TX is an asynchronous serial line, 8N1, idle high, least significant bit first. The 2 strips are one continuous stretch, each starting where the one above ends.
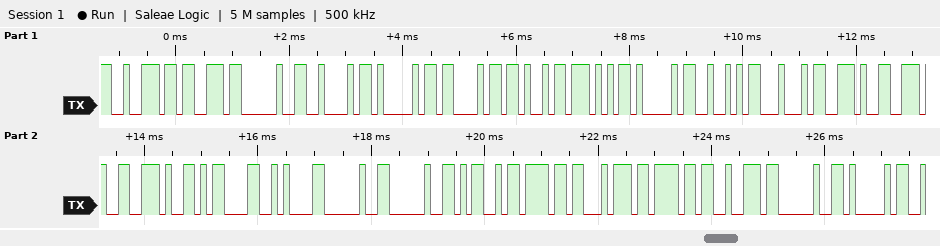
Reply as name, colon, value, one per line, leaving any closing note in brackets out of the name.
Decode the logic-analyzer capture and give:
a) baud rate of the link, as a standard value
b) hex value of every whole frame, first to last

baud rate of the link, as a standard value: 9600 baud
hex value of every whole frame, first to last: 72 73 20 42 41 43 4B 57 41 52 44 2E 2E 2E 0D 0A 20 20 4D 6F 74 6F 72 20 41
